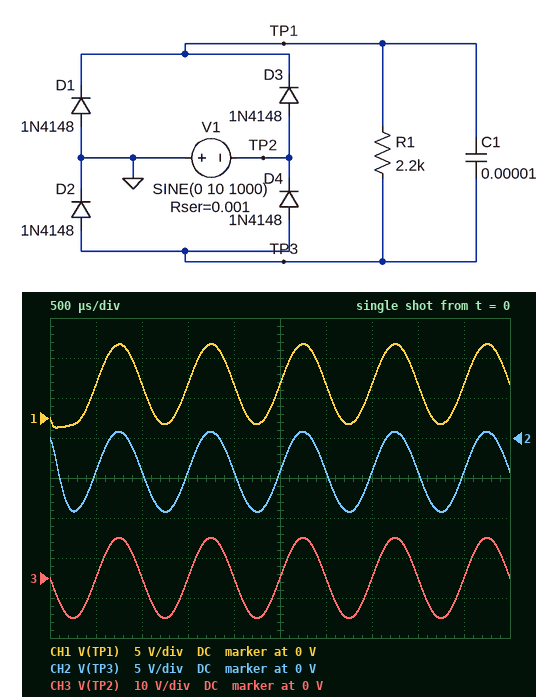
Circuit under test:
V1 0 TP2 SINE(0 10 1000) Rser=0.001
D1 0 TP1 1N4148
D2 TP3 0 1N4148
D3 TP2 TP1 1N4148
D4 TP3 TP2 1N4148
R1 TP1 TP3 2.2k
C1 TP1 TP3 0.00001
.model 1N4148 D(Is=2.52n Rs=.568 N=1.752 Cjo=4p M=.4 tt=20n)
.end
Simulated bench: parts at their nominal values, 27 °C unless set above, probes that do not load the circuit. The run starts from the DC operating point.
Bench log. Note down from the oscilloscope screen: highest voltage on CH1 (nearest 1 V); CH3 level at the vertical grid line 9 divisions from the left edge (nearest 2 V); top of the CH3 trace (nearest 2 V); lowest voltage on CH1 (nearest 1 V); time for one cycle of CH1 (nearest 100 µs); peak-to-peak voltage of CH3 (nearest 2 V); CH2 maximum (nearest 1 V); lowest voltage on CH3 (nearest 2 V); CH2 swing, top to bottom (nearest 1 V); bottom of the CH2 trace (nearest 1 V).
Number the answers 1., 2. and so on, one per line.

1. 9 V
2. 0 V
3. 10 V
4. -1 V
5. 1.0 ms
6. 20 V
7. 1 V
8. -10 V
9. 10 V
10. -9 V
